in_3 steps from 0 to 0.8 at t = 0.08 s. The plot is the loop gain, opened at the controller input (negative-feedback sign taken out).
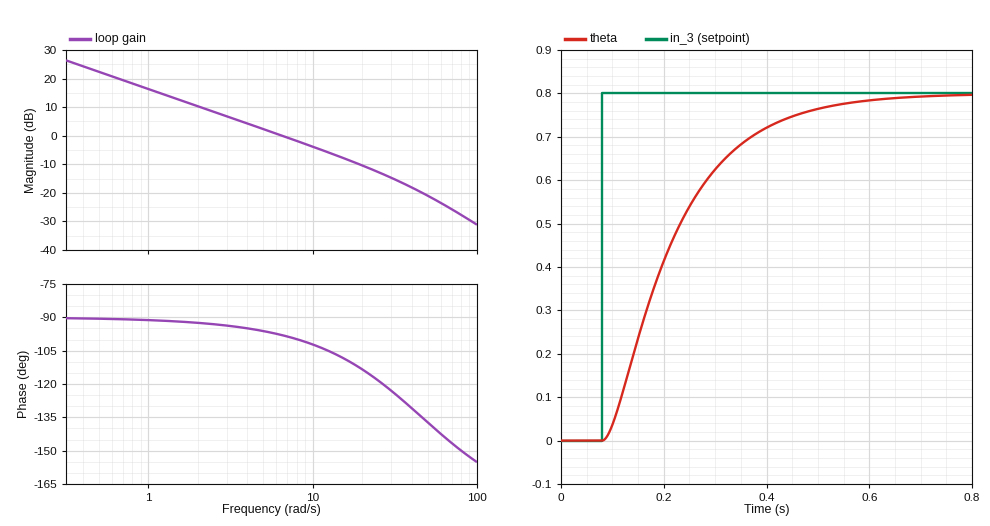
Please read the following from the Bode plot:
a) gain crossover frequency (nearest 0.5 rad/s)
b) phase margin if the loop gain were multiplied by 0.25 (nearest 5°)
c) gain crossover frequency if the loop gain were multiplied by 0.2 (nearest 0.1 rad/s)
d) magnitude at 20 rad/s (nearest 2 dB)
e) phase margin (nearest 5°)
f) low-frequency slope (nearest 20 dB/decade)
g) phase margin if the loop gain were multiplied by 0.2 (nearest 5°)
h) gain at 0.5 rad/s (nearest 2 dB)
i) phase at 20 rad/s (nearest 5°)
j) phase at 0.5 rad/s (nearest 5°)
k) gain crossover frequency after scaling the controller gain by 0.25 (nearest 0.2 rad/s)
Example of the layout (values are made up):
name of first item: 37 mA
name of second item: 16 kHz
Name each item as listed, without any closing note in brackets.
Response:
gain crossover frequency: 6.5 rad/s
phase margin if the loop gain were multiplied by 0.25: 90°
gain crossover frequency if the loop gain were multiplied by 0.2: 1.3 rad/s
magnitude at 20 rad/s: -10 dB
phase margin: 80°
low-frequency slope: -20 dB/decade
phase margin if the loop gain were multiplied by 0.2: 90°
gain at 0.5 rad/s: 22 dB
phase at 20 rad/s: -115°
phase at 0.5 rad/s: -90°
gain crossover frequency after scaling the controller gain by 0.25: 1.6 rad/s
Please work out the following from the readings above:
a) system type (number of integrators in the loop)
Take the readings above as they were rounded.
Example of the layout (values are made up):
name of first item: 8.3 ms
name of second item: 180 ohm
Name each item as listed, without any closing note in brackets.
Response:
system type: 1
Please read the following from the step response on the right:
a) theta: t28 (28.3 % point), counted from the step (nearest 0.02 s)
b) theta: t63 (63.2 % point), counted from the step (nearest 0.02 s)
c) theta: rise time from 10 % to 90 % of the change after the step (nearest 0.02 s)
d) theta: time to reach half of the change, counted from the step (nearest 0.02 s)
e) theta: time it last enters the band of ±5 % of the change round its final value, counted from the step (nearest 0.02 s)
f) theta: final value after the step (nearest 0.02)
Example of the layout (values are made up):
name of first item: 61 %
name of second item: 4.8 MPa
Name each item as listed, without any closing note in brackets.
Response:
theta: t28 (28.3 % point), counted from the step: 0.06 s
theta: t63 (63.2 % point), counted from the step: 0.16 s
theta: rise time from 10 % to 90 % of the change after the step: 0.28 s
theta: time to reach half of the change, counted from the step: 0.12 s
theta: time it last enters the band of ±5 % of the change round its final value, counted from the step: 0.40 s
theta: final value after the step: 0.80
